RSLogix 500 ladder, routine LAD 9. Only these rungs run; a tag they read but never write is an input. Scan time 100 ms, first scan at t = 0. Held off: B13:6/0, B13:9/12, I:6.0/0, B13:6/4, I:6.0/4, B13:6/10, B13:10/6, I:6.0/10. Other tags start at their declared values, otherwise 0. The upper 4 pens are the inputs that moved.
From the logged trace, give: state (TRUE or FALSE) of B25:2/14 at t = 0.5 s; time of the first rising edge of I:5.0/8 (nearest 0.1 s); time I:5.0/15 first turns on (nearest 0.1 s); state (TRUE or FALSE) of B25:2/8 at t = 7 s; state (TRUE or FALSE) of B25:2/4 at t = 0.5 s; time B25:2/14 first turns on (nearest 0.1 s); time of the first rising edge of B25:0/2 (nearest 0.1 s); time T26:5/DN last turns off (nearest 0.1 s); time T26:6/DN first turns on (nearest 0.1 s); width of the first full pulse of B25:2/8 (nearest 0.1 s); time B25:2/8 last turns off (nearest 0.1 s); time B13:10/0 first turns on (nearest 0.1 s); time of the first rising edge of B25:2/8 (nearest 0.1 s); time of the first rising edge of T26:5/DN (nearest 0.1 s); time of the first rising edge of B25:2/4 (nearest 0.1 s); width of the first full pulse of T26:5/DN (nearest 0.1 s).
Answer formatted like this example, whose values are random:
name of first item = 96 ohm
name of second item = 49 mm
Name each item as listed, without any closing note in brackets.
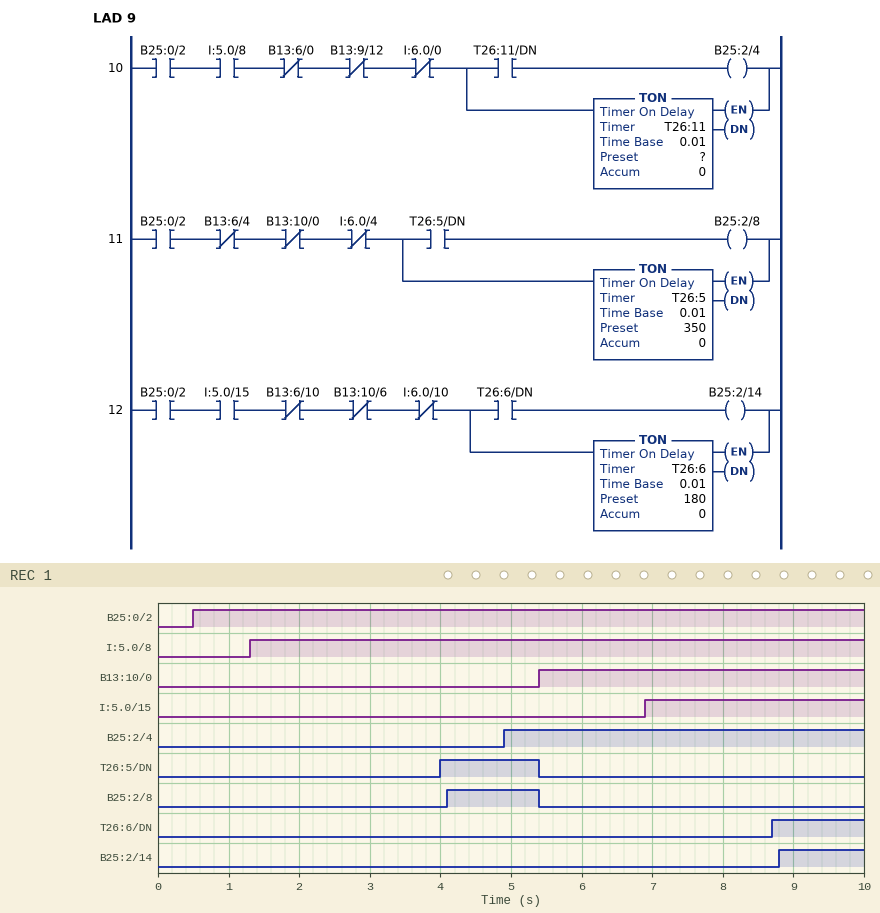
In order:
state (TRUE or FALSE) of B25:2/14 at t = 0.5 s = FALSE
time of the first rising edge of I:5.0/8 = 1.3 s
time I:5.0/15 first turns on = 6.9 s
state (TRUE or FALSE) of B25:2/8 at t = 7 s = FALSE
state (TRUE or FALSE) of B25:2/4 at t = 0.5 s = FALSE
time B25:2/14 first turns on = 8.8 s
time of the first rising edge of B25:0/2 = 0.5 s
time T26:5/DN last turns off = 5.4 s
time T26:6/DN first turns on = 8.7 s
width of the first full pulse of B25:2/8 = 1.3 s
time B25:2/8 last turns off = 5.4 s
time B13:10/0 first turns on = 5.4 s
time of the first rising edge of B25:2/8 = 4.1 s
time of the first rising edge of T26:5/DN = 4.0 s
time of the first rising edge of B25:2/4 = 4.9 s
width of the first full pulse of T26:5/DN = 1.4 s
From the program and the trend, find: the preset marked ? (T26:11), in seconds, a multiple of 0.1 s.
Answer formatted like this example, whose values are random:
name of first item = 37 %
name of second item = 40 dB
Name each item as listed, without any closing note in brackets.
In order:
the preset marked ? (T26:11), in seconds, a multiple of 0.1 s = 3.5 s
